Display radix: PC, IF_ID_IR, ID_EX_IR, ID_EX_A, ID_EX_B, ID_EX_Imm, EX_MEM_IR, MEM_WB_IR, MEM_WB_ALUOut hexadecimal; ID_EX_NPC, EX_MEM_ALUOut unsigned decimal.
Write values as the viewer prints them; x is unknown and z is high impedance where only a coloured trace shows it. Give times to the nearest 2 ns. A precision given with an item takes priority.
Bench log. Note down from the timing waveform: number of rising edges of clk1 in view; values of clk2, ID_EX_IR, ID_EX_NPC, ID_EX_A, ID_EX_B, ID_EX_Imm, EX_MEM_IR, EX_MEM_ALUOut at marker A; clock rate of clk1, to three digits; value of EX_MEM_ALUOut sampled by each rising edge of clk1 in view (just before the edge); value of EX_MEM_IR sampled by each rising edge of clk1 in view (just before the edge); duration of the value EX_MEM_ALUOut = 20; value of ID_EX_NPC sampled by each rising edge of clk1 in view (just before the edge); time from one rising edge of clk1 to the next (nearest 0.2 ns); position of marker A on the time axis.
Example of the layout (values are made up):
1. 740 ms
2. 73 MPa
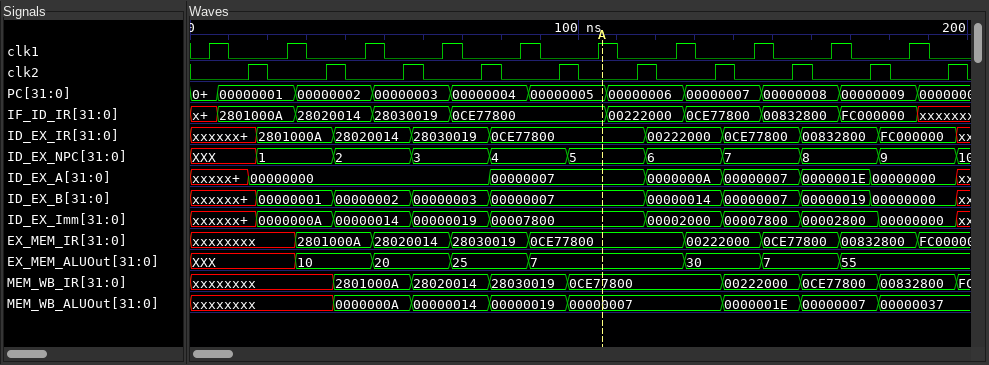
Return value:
1. 10
2. clk2=0, ID_EX_IR=0CE77800, ID_EX_NPC=5, ID_EX_A=00000007, ID_EX_B=00000007, ID_EX_Imm=00007800, EX_MEM_IR=0CE77800, EX_MEM_ALUOut=7
3. 50.0 MHz
4. XXX, XXX, 10, 20, 25, 7, 7, 30, 7, 55
5. xxxxxxxx, xxxxxxxx, 2801000A, 28020014, 28030019, 0CE77800, 0CE77800, 00222000, 0CE77800, 00832800
6. 20 ns
7. XXX, 1, 2, 3, 4, 5, 6, 7, 8, 9
8. 20 ns
9. 106 ns
